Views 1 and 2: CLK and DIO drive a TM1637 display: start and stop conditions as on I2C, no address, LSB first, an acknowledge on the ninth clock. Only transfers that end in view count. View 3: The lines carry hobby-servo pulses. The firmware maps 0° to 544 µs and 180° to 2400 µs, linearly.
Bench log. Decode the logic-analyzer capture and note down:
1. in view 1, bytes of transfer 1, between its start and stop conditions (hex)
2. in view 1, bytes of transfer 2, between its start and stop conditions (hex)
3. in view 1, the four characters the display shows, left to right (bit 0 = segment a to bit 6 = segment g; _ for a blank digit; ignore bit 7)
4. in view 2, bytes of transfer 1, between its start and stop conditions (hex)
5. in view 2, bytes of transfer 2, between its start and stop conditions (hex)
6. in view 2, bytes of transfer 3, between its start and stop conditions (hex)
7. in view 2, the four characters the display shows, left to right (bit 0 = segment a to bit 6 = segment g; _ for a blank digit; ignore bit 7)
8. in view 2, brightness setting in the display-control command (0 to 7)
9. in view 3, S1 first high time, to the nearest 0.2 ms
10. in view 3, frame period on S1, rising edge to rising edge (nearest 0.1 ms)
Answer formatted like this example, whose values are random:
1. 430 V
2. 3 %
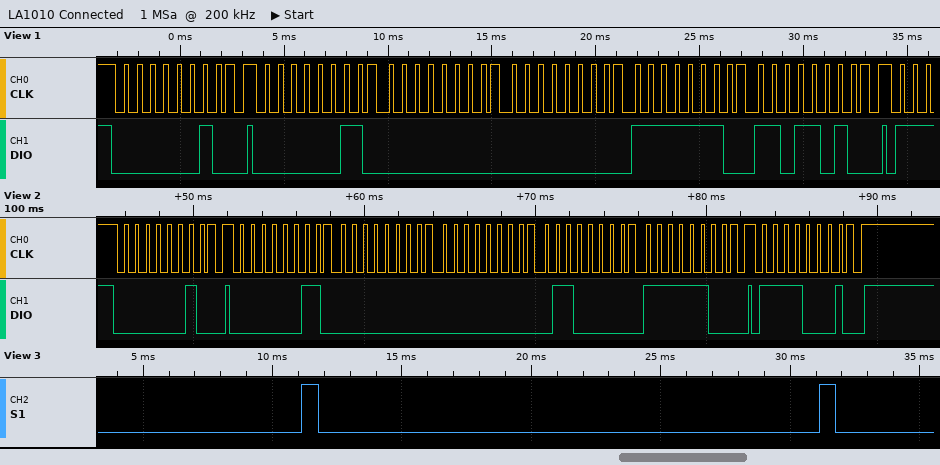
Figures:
1. 40
2. C0 00 00 7F 5B
3. __82
4. 40
5. C0 00 00 06 3F
6. 8F
7. __10
8. 7
9. 0.6 ms
10. 20.0 ms
